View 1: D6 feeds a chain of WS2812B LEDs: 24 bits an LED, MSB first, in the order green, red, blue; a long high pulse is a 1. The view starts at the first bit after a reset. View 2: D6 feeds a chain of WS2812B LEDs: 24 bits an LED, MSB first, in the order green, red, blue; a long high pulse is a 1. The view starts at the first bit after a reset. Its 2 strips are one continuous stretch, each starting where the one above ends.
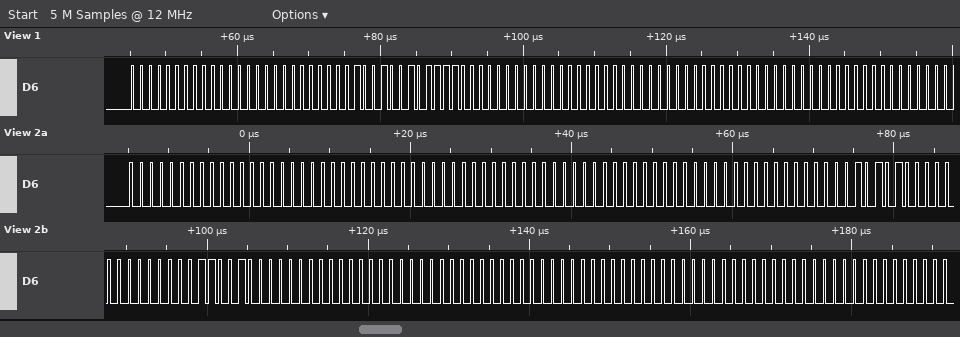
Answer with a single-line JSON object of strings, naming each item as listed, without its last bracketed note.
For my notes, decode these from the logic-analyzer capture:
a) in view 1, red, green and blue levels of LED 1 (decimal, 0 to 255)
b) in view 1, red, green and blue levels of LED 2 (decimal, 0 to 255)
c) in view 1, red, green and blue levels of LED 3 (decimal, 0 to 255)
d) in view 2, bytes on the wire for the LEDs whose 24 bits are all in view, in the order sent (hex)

{"in view 1, red, green and blue levels of LED 1": "0, 0, 0", "in view 1, red, green and blue levels of LED 2": "120, 73, 0", "in view 1, red, green and blue levels of LED 3": "0, 0, 0", "in view 2, bytes on the wire for the LEDs whose 24 bits are all in view, in the order sent": "00 00 00 00 00 00 00 00 00 A8 00 19 00 00 00 00 00 00"}
